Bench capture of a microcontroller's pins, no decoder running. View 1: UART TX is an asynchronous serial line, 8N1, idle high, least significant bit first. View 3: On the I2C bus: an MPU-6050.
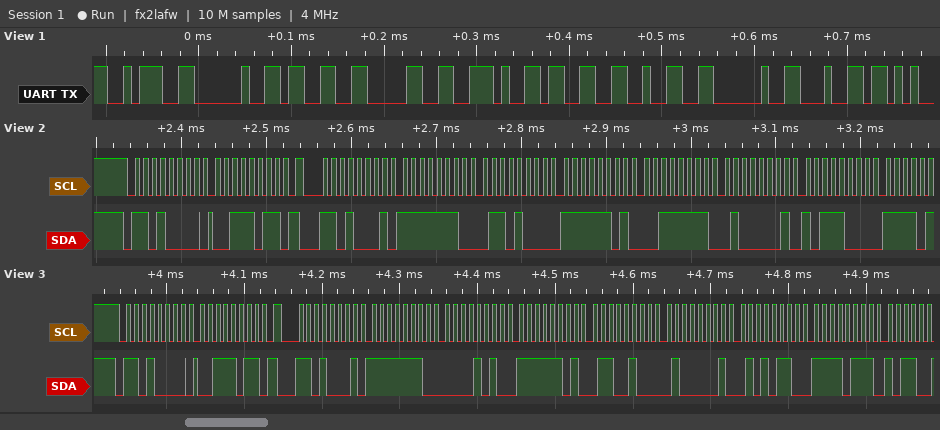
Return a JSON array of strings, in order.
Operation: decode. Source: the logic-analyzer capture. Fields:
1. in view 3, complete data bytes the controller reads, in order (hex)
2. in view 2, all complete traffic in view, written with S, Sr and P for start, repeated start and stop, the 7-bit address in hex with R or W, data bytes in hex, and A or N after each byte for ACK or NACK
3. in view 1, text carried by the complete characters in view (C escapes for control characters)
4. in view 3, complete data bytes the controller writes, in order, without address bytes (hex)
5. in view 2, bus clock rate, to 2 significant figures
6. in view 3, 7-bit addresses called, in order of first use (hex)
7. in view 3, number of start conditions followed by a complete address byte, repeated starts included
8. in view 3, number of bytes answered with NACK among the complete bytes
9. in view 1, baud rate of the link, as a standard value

["FE 0A FD 64 41 56 F7", "S 68W A 3B A Sr 68R A FE A 68 A FD A 3F A 41 A B8 A", "\": 30.32 d\"", "3B", "100 kHz", "0x68", "2", "0", "115200 baud"]
